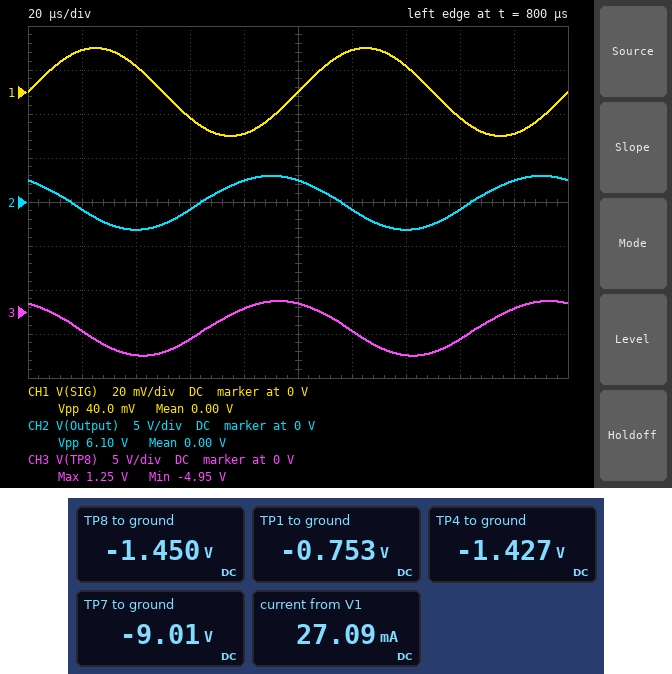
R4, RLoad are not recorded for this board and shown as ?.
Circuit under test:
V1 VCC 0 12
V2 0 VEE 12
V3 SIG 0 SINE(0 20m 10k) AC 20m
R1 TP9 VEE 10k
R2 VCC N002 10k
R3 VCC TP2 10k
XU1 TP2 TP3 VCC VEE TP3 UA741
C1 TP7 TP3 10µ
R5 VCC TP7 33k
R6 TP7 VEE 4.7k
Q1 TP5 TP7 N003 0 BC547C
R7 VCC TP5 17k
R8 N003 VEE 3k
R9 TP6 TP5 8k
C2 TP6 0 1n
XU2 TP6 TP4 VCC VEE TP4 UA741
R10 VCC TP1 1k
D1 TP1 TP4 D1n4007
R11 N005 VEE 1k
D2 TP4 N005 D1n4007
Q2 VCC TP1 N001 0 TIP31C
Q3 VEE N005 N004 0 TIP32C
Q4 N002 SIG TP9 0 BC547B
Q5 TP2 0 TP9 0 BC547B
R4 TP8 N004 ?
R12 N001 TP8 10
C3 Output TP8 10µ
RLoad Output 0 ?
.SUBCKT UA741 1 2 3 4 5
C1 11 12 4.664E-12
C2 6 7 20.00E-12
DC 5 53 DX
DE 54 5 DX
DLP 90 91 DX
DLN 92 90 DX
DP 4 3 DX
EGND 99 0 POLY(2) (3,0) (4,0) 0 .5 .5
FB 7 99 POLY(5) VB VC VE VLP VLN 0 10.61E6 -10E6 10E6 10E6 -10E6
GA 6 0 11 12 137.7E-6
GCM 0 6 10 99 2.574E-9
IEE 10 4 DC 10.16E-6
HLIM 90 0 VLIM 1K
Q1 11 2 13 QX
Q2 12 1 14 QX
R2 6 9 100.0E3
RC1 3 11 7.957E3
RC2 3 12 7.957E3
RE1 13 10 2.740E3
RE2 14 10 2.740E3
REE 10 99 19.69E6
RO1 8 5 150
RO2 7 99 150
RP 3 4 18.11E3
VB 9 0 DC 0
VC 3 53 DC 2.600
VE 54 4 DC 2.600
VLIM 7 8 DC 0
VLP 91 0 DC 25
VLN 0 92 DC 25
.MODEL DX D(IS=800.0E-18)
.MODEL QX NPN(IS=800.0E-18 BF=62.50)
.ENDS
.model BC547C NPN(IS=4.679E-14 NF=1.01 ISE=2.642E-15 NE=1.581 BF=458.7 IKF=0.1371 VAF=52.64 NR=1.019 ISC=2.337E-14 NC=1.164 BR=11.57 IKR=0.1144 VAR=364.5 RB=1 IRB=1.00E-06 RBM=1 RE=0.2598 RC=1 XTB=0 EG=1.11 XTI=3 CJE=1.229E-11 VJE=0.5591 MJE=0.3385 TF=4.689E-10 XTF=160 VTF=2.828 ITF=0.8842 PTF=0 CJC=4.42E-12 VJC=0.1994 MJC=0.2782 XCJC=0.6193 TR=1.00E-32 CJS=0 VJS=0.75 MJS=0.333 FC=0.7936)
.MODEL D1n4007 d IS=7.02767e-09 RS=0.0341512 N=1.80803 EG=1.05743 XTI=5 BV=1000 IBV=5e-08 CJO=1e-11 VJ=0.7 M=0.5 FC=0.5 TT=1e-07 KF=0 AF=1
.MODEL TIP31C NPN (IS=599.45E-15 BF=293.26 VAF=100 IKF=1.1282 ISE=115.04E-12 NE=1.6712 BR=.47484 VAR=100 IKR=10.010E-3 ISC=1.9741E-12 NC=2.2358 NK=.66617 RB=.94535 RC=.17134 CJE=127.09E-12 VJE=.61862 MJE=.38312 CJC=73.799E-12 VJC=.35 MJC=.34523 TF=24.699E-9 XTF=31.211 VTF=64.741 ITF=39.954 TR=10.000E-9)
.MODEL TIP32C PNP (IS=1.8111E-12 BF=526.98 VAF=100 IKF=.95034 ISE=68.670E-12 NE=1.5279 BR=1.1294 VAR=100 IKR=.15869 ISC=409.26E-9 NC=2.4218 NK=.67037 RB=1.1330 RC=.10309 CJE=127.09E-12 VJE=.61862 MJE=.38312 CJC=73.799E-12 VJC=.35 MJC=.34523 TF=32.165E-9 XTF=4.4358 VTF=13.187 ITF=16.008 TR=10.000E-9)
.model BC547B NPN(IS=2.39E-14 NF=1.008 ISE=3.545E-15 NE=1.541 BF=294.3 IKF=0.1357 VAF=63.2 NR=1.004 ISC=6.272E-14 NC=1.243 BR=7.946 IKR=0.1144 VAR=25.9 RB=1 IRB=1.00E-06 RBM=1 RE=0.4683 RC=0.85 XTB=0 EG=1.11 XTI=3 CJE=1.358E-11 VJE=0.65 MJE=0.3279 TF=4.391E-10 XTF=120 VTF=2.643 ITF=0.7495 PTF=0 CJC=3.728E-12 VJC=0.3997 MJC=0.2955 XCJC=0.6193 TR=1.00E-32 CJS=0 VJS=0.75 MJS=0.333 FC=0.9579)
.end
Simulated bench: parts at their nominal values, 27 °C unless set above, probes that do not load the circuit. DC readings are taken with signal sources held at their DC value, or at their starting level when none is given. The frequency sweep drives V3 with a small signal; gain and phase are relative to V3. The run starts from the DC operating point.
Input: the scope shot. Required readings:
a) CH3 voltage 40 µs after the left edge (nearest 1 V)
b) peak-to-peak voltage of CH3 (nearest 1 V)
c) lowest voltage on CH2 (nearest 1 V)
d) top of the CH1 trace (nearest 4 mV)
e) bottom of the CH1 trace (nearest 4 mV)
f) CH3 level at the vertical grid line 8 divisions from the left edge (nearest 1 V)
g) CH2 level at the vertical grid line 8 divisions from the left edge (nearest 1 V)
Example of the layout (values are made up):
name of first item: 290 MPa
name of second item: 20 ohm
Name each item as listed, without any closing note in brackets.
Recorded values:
CH3 voltage 40 µs after the left edge: -5 V
peak-to-peak voltage of CH3: 6 V
lowest voltage on CH2: -3 V
top of the CH1 trace: 20 mV
bottom of the CH1 trace: -20 mV
CH3 level at the vertical grid line 8 divisions from the left edge: -3 V
CH2 level at the vertical grid line 8 divisions from the left edge: -1 V
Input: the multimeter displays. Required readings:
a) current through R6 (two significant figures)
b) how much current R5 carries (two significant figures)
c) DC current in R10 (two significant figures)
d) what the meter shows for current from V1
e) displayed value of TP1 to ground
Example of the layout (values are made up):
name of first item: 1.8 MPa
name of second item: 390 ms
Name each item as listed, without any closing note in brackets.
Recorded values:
current through R6: 640 µA
how much current R5 carries: 640 µA
DC current in R10: 13 mA
what the meter shows for current from V1: 27.09 mA
displayed value of TP1 to ground: -0.753 V
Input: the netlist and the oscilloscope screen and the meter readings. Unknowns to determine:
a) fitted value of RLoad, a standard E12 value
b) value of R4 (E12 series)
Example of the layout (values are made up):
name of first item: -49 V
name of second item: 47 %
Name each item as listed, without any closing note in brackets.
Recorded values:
fitted value of RLoad, a standard E12 value: 10 Ω
value of R4: 6.8 Ω
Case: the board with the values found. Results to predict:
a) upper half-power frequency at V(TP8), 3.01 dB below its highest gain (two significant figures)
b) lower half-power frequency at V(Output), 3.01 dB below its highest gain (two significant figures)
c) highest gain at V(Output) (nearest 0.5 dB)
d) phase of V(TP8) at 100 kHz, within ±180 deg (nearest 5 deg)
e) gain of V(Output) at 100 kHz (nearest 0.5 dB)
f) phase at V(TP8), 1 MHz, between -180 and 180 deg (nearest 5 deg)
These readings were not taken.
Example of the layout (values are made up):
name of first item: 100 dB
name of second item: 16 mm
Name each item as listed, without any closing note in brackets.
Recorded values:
upper half-power frequency at V(TP8), 3.01 dB below its highest gain: 1.9 kHz
lower half-power frequency at V(Output), 3.01 dB below its highest gain: 800 Hz
highest gain at V(Output): 49.5 dB
phase of V(TP8) at 100 kHz, within ±180 deg: 80 deg
gain of V(Output) at 100 kHz: 27.0 dB
phase at V(TP8), 1 MHz, between -180 and 180 deg: -125 deg
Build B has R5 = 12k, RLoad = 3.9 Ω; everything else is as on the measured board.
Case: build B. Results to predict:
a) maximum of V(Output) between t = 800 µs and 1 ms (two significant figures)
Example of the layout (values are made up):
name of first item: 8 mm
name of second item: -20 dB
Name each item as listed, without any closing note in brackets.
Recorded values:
maximum of V(Output) between t = 800 µs and 1 ms: 240 mV
